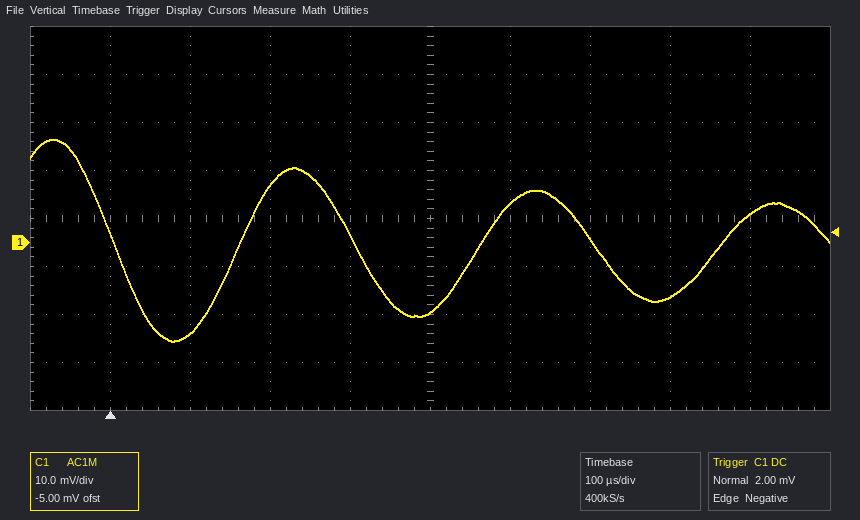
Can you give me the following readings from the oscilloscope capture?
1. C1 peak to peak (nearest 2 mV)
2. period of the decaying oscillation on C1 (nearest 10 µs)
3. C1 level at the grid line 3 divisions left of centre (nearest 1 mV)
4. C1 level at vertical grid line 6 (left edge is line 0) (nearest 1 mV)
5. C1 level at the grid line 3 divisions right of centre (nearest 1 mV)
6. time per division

42 mV
300 µs
-19 mV
8 mV
-11 mV
100 µs
